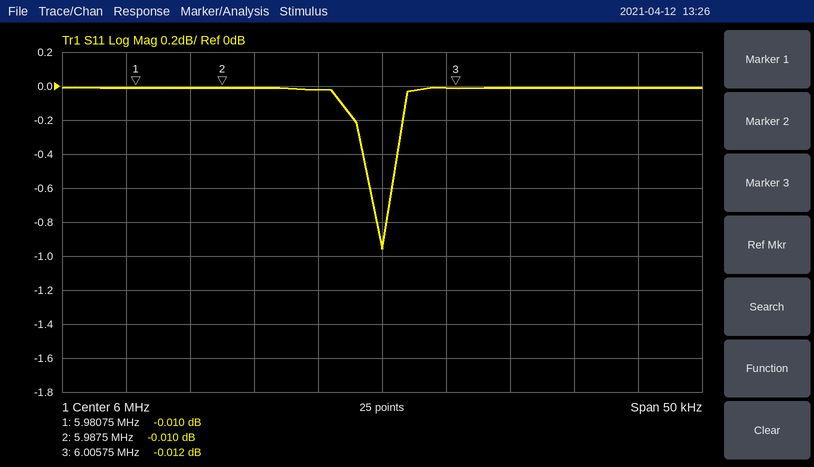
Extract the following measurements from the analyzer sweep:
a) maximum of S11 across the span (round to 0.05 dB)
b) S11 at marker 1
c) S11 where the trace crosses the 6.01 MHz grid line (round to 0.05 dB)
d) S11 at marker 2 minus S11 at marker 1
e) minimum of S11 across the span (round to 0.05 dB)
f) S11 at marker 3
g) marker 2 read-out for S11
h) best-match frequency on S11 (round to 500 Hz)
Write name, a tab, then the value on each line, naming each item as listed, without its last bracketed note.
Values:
maximum of S11 across the span	0.00 dB
S11 at marker 1	-0.010 dB
S11 where the trace crosses the 6.01 MHz grid line	0.00 dB
S11 at marker 2 minus S11 at marker 1	0.000 dB
minimum of S11 across the span	-0.95 dB
S11 at marker 3	-0.012 dB
marker 2 read-out for S11	-0.010 dB
best-match frequency on S11	6.0000 MHz
